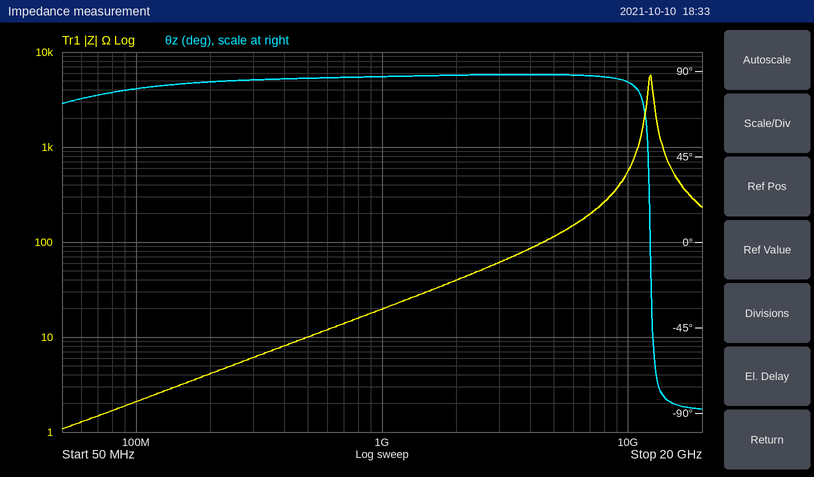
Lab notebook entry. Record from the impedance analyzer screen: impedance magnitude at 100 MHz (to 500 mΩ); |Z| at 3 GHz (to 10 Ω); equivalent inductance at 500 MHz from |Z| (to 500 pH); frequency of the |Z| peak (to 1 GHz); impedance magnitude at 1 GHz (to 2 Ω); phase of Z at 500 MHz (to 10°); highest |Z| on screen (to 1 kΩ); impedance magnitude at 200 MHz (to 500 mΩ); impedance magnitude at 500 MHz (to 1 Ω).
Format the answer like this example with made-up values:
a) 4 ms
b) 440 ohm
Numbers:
a) 2.0 Ω
b) 60 Ω
c) 3.0 nH
d) 12 GHz
e) 20 Ω
f) 90°
g) 6 kΩ
h) 4.0 Ω
i) 10 Ω
